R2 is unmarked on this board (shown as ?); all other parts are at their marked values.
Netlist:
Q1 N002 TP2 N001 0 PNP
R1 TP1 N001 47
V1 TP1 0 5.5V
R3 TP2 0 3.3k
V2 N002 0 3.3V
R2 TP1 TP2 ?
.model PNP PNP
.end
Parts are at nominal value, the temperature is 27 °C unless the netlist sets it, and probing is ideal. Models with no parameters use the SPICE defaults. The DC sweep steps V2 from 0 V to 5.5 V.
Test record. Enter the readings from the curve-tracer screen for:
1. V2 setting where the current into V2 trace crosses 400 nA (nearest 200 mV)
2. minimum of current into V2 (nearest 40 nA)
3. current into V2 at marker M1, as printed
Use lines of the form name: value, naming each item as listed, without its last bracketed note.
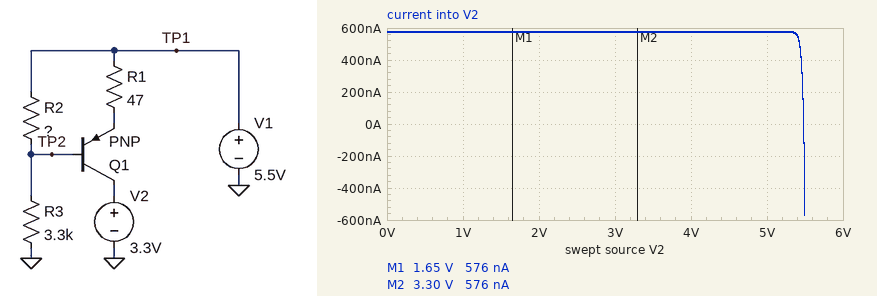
V2 setting where the current into V2 trace crosses 400 nA: 5.4 V
minimum of current into V2: -560 nA
current into V2 at marker M1, as printed: 576 nA
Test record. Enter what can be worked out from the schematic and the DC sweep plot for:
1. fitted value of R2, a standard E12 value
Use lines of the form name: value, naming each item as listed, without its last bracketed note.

fitted value of R2, a standard E12 value: 390 Ω
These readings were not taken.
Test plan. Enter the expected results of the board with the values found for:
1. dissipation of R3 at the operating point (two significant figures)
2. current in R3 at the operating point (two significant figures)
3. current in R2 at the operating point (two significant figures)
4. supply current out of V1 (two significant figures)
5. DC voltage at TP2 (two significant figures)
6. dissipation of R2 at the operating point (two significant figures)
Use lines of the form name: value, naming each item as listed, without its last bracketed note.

dissipation of R3 at the operating point: 7.3 mW
current in R3 at the operating point: 1.5 mA
current in R2 at the operating point: 1.5 mA
supply current out of V1: 1.5 mA
DC voltage at TP2: 4.9 V
dissipation of R2 at the operating point: 870 µW
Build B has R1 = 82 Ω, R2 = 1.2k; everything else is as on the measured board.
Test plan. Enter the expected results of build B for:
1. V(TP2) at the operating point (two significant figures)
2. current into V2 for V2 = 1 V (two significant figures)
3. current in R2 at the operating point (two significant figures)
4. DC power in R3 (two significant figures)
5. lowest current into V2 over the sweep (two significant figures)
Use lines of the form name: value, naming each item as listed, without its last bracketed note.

V(TP2) at the operating point: 4.1 V
current into V2 for V2 = 1 V: 7.0 mA
current in R2 at the operating point: 1.2 mA
DC power in R3: 5.1 mW
lowest current into V2 over the sweep: -790 µA
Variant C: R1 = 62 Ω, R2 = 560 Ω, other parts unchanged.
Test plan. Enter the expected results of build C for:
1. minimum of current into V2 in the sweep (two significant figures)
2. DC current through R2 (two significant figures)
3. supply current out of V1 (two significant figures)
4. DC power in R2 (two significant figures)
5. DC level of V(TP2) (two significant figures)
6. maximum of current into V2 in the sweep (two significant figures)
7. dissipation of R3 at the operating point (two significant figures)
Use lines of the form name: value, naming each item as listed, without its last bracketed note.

minimum of current into V2 in the sweep: -150 µA
DC current through R2: 1.4 mA
supply current out of V1: 2.0 mA
DC power in R2: 1.1 mW
DC level of V(TP2): 4.7 V
maximum of current into V2 in the sweep: 570 µA
dissipation of R3 at the operating point: 6.7 mW
